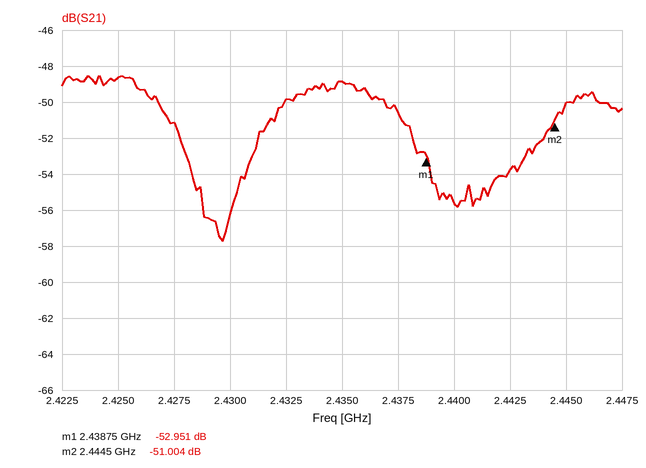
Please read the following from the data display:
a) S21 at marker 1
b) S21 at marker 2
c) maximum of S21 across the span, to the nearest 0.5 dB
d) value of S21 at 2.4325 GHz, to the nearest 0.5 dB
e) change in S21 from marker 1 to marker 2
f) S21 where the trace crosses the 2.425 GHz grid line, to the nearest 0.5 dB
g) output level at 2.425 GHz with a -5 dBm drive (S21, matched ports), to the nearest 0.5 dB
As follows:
-52.951 dB
-51.004 dB
-48.5 dB
-50.0 dB
1.947 dB
-48.5 dB
-53.5 dBm
